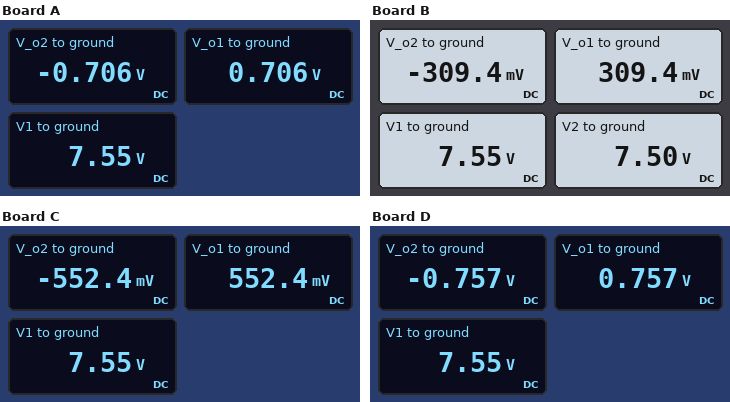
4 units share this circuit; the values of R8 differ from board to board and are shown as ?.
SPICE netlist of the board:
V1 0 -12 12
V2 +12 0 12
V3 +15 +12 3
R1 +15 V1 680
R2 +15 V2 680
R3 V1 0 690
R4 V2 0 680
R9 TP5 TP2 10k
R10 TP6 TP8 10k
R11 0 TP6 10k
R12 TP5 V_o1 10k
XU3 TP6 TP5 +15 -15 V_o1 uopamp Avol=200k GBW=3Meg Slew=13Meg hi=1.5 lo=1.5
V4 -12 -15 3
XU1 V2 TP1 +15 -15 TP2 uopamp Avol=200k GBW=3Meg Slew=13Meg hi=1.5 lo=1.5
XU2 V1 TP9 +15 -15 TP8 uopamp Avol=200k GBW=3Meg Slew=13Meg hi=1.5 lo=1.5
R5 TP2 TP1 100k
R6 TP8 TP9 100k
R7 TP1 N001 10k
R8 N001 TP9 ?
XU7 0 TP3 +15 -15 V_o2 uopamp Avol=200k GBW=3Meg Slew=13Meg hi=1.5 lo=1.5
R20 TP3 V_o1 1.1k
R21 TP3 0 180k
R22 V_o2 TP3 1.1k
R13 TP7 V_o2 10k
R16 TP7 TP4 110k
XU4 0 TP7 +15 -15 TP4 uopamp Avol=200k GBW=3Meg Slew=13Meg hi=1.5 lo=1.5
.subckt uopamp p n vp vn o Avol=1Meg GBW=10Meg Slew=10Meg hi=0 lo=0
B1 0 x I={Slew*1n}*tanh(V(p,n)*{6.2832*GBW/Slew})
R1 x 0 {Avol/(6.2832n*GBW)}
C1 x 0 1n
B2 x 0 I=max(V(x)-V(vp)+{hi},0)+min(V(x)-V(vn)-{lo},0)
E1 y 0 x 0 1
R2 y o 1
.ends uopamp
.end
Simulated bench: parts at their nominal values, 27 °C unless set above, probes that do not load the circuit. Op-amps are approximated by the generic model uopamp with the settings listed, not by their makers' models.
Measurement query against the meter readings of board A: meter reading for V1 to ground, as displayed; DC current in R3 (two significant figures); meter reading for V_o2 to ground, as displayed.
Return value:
7.55 V
11 mA
-0.706 V
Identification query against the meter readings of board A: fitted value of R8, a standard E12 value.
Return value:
6.8 kΩ
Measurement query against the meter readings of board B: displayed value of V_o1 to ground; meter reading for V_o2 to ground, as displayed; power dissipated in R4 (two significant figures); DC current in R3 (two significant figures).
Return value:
309.4 mV
-309.4 mV
83 mW
11 mA
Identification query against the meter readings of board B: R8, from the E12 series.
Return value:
33 kΩ
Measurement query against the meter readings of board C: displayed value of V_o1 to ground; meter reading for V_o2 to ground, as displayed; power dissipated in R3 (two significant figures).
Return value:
552.4 mV
-552.4 mV
83 mW
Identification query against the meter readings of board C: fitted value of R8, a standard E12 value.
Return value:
12 kΩ
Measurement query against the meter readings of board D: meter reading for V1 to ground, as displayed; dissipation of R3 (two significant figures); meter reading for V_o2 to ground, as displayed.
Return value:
7.55 V
83 mW
-0.757 V
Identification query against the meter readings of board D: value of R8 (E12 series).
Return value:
5.6 kΩ
